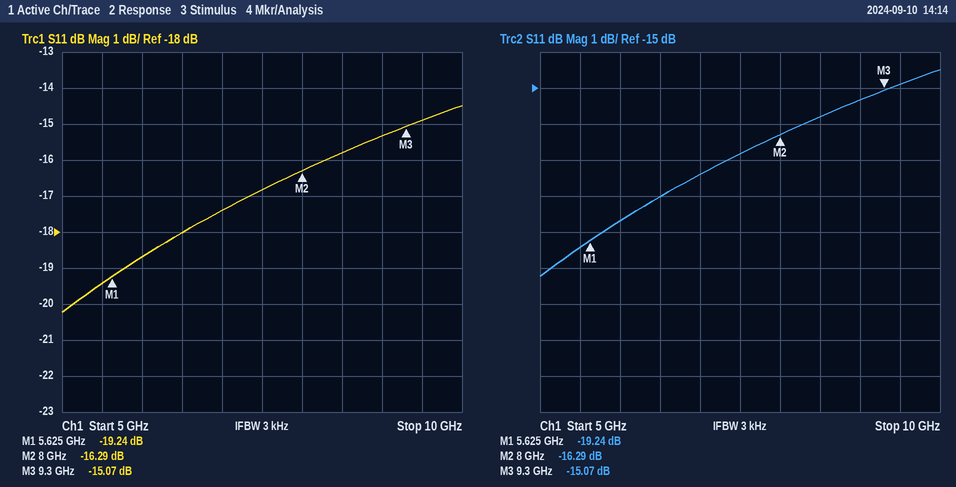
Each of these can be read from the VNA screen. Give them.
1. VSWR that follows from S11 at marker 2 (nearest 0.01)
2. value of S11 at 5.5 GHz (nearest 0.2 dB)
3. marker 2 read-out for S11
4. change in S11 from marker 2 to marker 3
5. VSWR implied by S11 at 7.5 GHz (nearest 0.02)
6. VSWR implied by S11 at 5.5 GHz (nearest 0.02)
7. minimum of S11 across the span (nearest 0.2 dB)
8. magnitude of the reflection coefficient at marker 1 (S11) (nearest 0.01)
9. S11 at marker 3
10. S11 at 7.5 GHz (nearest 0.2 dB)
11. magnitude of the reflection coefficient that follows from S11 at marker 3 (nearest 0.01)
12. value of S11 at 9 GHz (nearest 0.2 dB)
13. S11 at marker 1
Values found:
1.36
-19.4 dB
-16.29 dB
1.22 dB
1.34
1.24
-20.2 dB
0.11
-15.07 dB
-16.8 dB
0.18
-15.4 dB
-19.24 dB
